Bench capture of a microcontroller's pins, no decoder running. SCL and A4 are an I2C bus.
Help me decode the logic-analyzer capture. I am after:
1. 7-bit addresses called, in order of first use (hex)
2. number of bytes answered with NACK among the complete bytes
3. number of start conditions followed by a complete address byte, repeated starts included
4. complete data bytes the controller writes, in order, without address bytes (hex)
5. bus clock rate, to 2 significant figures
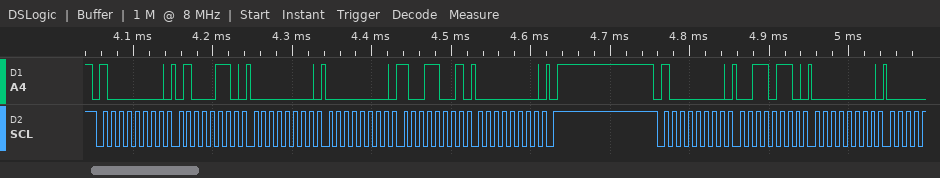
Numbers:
0x40
0
2
46 00 00 99 00 36 00
100 kHz
